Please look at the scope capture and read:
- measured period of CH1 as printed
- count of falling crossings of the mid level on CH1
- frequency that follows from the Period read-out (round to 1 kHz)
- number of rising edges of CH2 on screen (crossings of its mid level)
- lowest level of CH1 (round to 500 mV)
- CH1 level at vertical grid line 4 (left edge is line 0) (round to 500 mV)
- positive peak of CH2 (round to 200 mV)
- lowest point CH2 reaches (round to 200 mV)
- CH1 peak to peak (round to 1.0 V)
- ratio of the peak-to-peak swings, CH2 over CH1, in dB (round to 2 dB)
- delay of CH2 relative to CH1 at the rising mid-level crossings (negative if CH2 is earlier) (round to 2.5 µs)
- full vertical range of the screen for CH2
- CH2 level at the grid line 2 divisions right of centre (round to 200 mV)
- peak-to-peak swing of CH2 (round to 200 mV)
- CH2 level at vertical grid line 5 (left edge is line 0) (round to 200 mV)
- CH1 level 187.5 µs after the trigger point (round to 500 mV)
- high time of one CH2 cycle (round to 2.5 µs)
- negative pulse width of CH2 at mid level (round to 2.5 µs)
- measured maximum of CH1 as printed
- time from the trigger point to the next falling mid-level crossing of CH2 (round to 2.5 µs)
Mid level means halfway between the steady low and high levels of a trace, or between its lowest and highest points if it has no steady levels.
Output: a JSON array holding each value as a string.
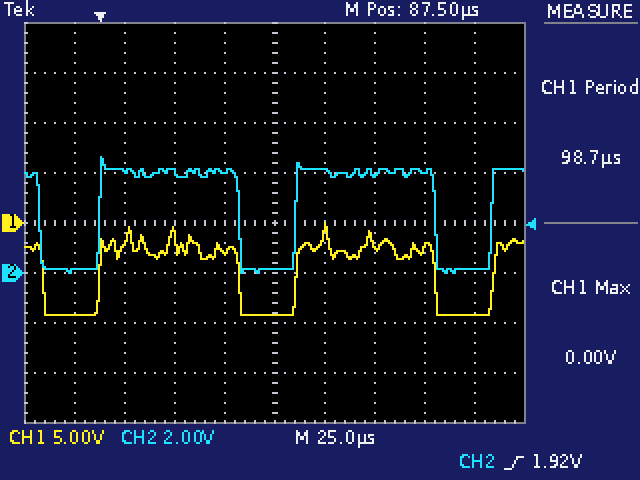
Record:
["98.7 µs", "3", "10 kHz", "3", "-9.0 V", "-3.0 V", "4.6 V", "0.0 V", "9.0 V", "-6 dB", "0.0 µs", "16 V", "4.0 V", "4.6 V", "200 mV", "-9.0 V", "70.0 µs", "27.5 µs", "0.00 V", "70.0 µs"]
